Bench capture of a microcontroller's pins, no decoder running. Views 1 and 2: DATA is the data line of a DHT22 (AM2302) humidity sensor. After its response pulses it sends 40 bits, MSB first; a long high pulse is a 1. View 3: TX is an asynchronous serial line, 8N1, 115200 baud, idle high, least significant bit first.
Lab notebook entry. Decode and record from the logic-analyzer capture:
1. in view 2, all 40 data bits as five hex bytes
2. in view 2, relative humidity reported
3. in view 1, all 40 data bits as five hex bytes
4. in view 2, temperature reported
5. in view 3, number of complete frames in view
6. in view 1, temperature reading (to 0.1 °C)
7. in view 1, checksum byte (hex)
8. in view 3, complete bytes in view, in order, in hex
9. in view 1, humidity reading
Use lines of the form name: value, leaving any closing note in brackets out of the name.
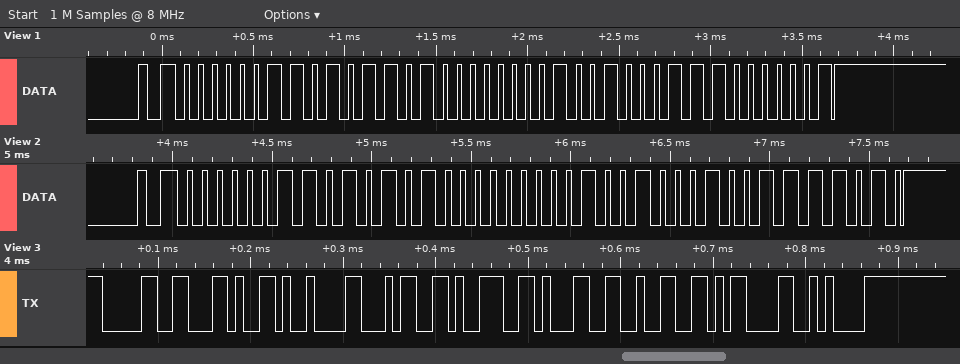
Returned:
in view 2, all 40 data bits as five hex bytes: 03 54 01 22 7A
in view 2, relative humidity reported: 85.2 %
in view 1, all 40 data bits as five hex bytes: 03 5A 01 23 81
in view 2, temperature reported: 29.0 °C
in view 3, number of complete frames in view: 9
in view 1, temperature reading: 29.1 °C
in view 1, checksum byte: 0x81
in view 3, complete bytes in view, in order, in hex: 30 2C 09 34 39 31 32 0D 0A
in view 1, humidity reading: 85.8 %
